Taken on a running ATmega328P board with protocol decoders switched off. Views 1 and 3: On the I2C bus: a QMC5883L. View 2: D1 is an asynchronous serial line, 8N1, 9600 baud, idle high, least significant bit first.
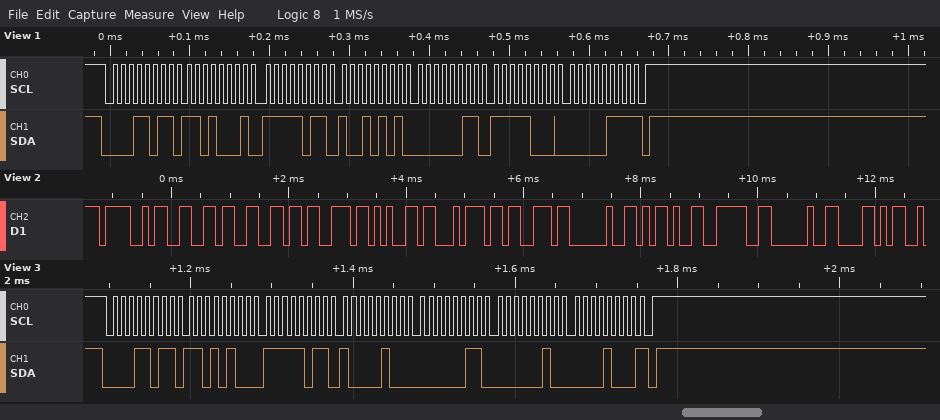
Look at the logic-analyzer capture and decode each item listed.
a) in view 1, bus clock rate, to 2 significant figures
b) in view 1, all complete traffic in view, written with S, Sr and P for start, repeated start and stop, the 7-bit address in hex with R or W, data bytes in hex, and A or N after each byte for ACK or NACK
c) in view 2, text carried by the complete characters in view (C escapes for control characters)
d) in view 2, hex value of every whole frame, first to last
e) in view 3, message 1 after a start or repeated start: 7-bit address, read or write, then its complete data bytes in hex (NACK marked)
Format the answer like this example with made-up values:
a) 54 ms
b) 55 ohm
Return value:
a) 100 kHz
b) S 0DR A D1 A FB A 95 A 03 A F8 A 07 N P
c) "Offsets -> X"
d) 4F 66 66 73 65 74 73 20 2D 3E 20 58
e) 0x0D read: D4 FB 84 03 02 08 NACK
